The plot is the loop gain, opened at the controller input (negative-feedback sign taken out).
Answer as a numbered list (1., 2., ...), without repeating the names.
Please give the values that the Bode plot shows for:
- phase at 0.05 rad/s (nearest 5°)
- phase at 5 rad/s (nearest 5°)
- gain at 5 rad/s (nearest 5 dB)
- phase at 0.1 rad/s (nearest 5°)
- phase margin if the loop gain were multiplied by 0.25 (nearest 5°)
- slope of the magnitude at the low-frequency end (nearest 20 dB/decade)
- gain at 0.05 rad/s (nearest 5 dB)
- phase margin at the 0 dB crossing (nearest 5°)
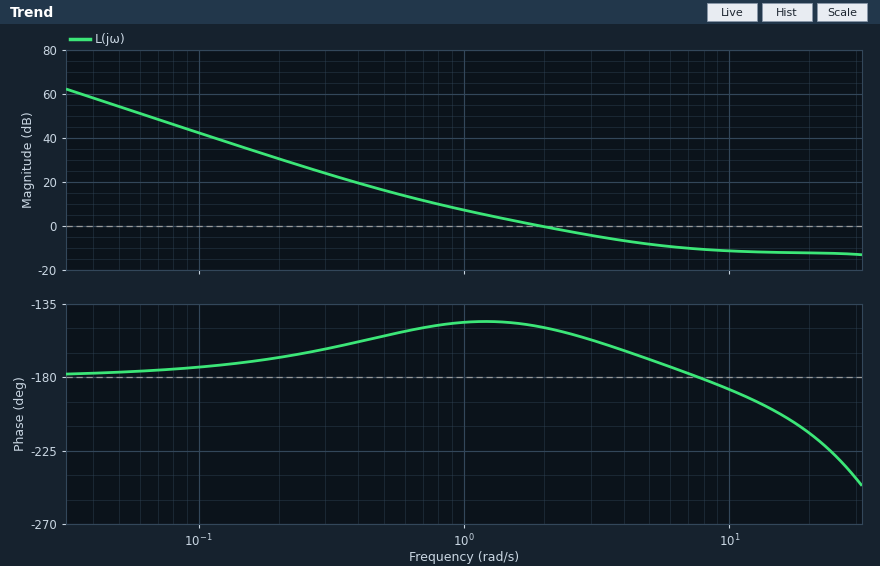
1. -175°
2. -170°
3. -10 dB
4. -175°
5. 30°
6. -40 dB/decade
7. 55 dB
8. 30°
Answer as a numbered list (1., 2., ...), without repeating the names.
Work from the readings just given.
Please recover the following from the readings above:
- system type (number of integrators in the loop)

1. 2
